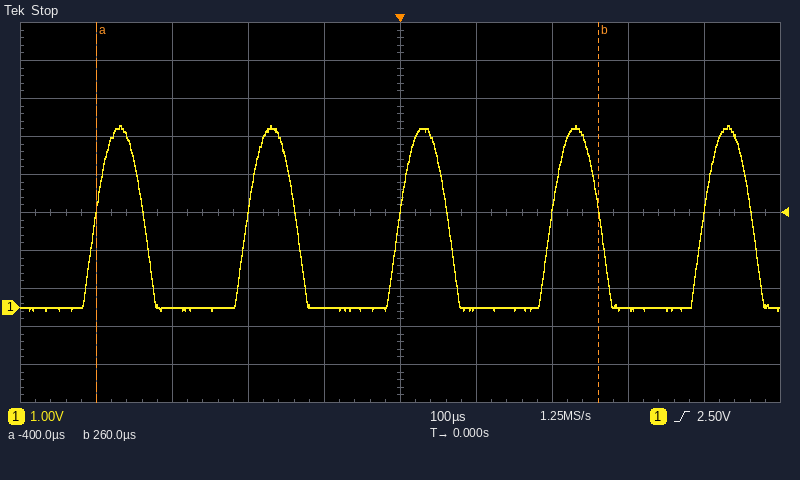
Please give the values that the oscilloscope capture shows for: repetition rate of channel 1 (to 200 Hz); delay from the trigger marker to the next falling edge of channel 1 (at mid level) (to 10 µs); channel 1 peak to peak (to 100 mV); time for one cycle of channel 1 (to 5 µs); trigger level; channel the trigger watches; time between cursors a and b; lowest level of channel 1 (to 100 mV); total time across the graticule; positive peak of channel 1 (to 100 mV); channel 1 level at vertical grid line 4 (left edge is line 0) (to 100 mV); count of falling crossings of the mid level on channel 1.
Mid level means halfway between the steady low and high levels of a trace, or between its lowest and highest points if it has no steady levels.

5.0 kHz
60 µs
4.9 V
200 µs
2.50 V
channel 1
660 µs
-100 mV
1 ms
4.8 V
0.0 V
5
